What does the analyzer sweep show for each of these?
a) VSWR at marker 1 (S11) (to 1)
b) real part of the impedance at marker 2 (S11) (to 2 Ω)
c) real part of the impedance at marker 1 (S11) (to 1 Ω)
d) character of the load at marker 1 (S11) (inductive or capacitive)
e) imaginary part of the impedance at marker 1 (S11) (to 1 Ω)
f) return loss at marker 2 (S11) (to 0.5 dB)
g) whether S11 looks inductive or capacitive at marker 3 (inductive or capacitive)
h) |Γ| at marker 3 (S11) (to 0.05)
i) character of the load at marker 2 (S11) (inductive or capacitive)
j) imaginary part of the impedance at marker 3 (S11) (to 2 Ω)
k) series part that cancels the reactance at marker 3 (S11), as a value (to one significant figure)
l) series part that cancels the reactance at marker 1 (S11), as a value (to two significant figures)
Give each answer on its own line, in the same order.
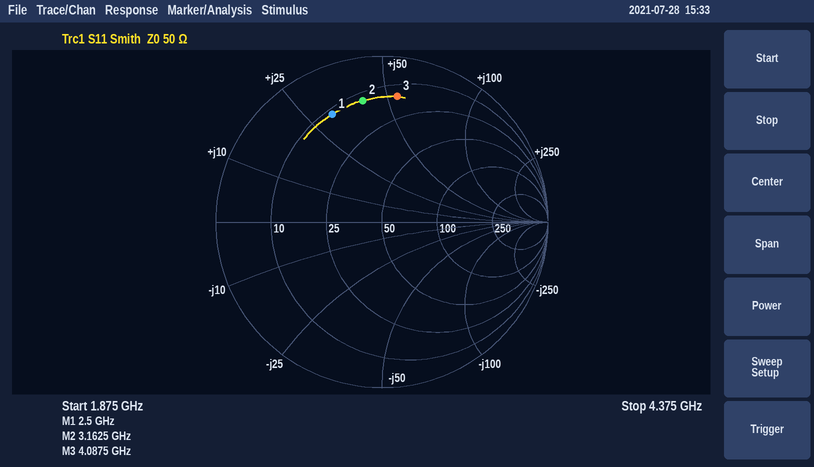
6
12 Ω
12 Ω
inductive
+31 Ω
2.5 dB
inductive
0.75
inductive
+54 Ω
700 fF
2.1 pF
